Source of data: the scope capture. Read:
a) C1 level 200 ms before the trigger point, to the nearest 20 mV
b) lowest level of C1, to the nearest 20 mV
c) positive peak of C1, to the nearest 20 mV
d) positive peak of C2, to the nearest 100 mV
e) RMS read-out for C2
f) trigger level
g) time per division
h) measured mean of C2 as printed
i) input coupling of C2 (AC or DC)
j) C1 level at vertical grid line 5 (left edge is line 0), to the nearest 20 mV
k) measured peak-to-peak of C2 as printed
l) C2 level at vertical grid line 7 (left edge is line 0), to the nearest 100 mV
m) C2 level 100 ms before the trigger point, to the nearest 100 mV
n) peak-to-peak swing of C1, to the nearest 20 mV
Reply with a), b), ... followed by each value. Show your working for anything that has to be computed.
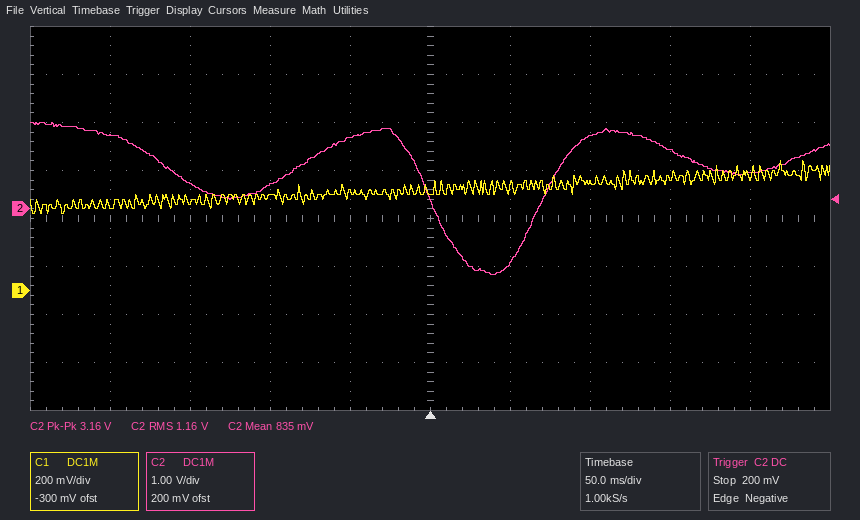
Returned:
a) 360 mV
b) 320 mV
c) 540 mV
d) 1.8 V
e) 1.16 V
f) 200 mV
g) 50 ms
h) 835 mV
i) DC
j) 420 mV
k) 3.16 V
l) 1.5 V
m) 500 mV
n) 540 mV − (320 mV) = 220 mV
